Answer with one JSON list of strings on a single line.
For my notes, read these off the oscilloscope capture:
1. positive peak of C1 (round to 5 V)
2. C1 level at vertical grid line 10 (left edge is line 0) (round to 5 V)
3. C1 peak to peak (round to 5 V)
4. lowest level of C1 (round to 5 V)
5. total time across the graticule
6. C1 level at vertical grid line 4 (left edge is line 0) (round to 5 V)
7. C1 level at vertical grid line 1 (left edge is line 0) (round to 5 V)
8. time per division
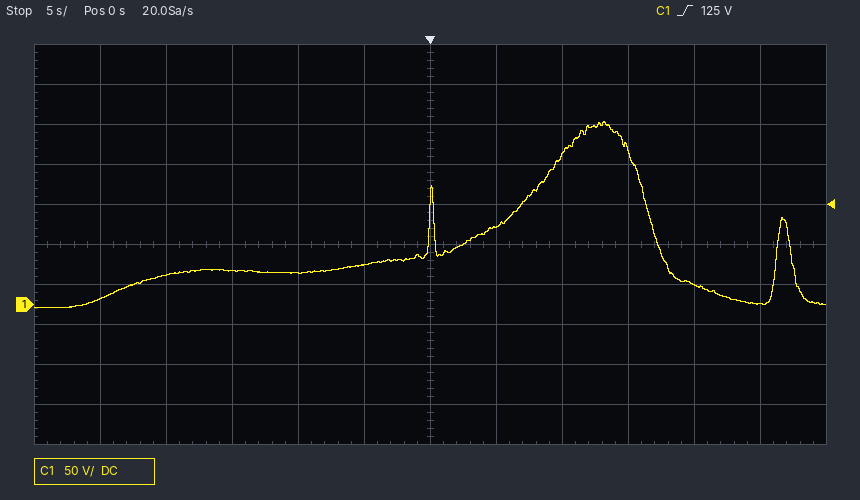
["230 V", "25 V", "235 V", "-5 V", "60 s", "40 V", "5 V", "5 s"]
